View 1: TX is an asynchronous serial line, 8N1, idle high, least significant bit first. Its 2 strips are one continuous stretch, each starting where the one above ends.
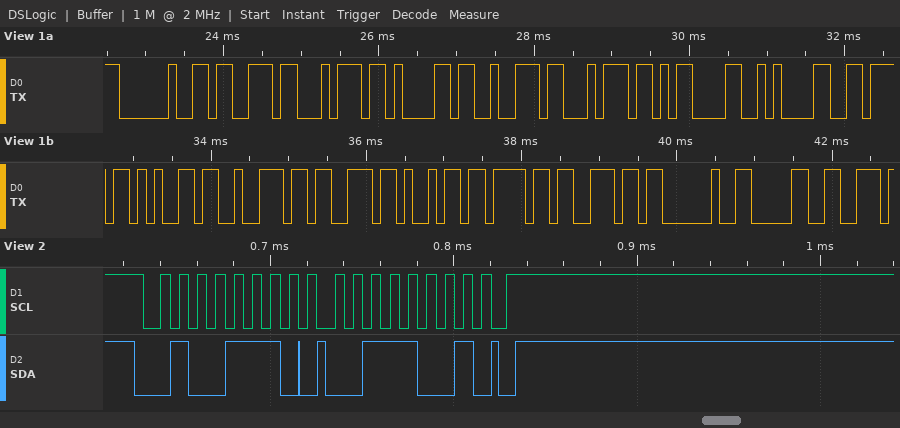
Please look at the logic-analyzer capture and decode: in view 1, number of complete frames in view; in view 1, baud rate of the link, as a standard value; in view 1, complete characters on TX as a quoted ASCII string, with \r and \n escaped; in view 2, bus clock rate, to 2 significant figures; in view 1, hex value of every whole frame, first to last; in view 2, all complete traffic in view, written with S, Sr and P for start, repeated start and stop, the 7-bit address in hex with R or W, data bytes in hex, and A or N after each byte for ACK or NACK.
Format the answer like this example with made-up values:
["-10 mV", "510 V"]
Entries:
["17", "9600 baud", "\" start\\r\\nversion 0\"", "100 kHz", "0x20 0x73 0x74 0x61 0x72 0x74 0x0D 0x0A 0x76 0x65 0x72 0x73 0x69 0x6F 0x6E 0x20 0x30", "S 27W A 39 A P"]
